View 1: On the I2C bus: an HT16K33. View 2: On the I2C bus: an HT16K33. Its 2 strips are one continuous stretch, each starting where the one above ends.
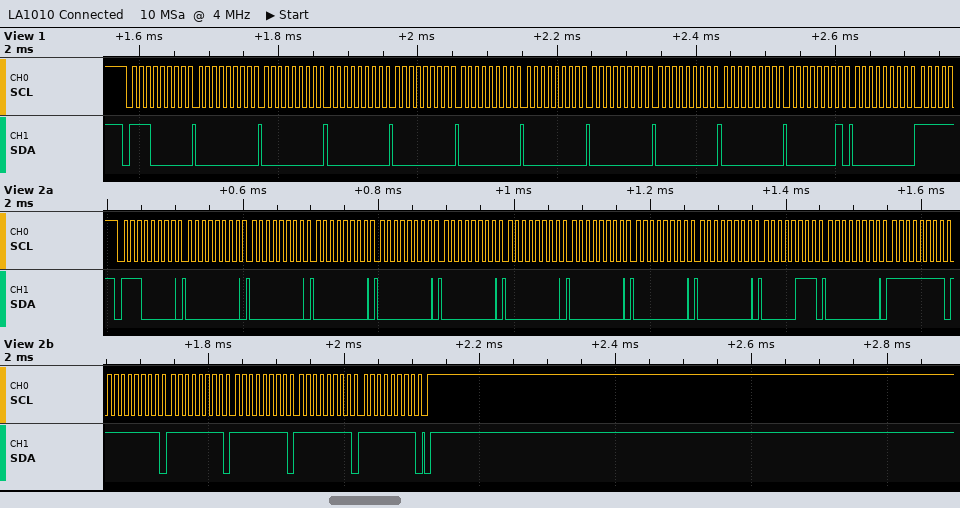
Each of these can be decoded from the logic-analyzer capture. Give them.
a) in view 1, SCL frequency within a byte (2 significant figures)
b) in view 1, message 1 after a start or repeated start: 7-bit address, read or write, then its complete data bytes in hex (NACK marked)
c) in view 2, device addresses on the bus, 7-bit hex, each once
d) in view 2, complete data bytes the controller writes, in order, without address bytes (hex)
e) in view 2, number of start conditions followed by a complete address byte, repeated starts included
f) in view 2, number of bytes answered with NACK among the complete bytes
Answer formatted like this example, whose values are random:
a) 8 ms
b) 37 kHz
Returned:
a) 100 kHz
b) 0x70 write: 00 00 00 00 00 00 00 00 00 01 00
c) 0x70
d) 00 00 00 00 00 00 00 00 00 07 00 FF FF FF FF FF FF
e) 1
f) 0
